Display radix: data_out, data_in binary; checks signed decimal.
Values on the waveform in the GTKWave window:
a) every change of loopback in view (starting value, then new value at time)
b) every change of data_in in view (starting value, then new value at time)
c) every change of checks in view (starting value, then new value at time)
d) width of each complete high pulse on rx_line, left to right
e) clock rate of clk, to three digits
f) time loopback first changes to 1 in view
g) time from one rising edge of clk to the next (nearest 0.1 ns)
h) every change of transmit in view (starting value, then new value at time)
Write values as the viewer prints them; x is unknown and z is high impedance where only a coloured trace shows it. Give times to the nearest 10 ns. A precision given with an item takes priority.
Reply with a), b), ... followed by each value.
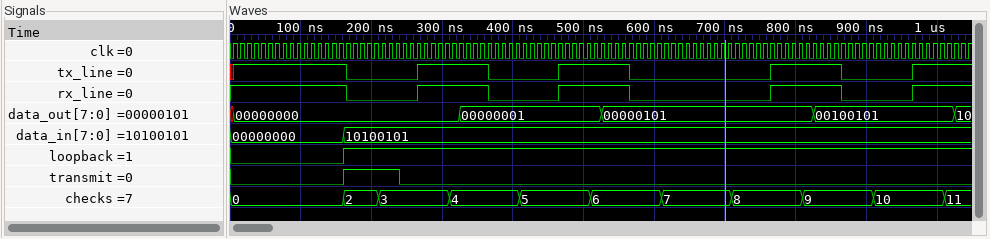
a) 0, 1 at 160 ns
b) 00000000, 10100101 at 160 ns
c) 0, 2 at 160 ns, 3 at 210 ns, 4 at 310 ns, 5 at 410 ns, 6 at 510 ns, 7 at 610 ns, 8 at 710 ns, 9 at 810 ns, 10 at 910 ns, 11 at 1010 ns
d) 100 ns, 100 ns, 100 ns
e) 100 MHz
f) 160 ns
g) 10 ns
h) 0, 1 at 160 ns, 0 at 240 ns
